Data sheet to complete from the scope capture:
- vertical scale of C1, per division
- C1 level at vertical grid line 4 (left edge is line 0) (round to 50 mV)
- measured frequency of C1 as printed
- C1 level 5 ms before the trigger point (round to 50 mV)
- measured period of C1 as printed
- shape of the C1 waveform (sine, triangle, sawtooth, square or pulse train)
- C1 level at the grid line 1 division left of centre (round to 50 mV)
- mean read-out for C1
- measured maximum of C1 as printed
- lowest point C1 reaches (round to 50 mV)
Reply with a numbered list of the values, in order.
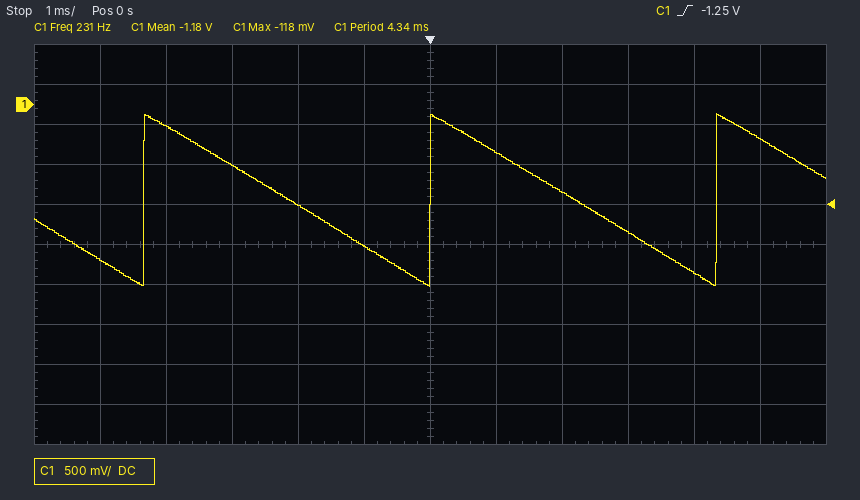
1. 500 mV
2. -1.25 V
3. 231 Hz
4. -1.95 V
5. 4.34 ms
6. sawtooth
7. -1.75 V
8. -1.18 V
9. -118 mV
10. -2.25 V
